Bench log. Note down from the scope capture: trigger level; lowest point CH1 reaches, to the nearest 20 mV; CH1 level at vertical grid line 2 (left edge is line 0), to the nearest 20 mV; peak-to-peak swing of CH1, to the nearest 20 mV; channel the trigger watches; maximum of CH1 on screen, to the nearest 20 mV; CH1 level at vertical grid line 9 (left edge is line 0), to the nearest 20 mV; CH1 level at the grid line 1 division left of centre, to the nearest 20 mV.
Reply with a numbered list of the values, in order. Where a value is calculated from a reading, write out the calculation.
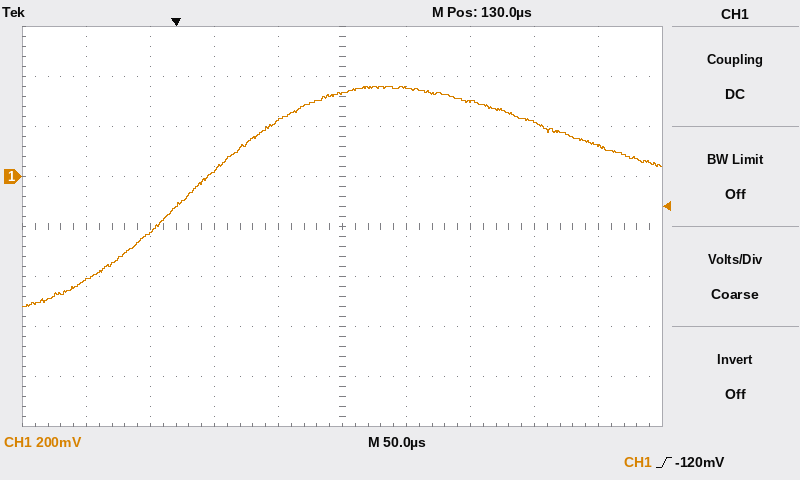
1. -120 mV
2. -520 mV
3. -220 mV
4. 360 mV − (-520 mV) = 880 mV
5. CH1
6. 360 mV
7. 120 mV
8. 220 mV
